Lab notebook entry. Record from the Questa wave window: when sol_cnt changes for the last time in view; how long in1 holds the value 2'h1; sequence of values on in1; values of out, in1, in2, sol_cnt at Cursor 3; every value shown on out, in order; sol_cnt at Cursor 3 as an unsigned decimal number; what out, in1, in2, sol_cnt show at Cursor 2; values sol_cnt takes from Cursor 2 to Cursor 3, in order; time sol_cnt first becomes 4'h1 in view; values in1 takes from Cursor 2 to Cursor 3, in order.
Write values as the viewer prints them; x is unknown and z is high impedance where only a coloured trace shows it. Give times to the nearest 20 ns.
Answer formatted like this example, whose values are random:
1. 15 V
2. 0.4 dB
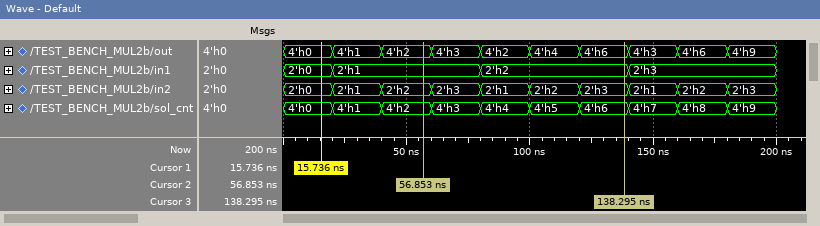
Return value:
1. 180 ns
2. 60 ns
3. 2'h0, 2'h1, 2'h2, 2'h3
4. out=4'h6, in1=2'h2, in2=2'h3, sol_cnt=4'h6
5. 4'h0, 4'h1, 4'h2, 4'h3, 4'h2, 4'h4, 4'h6, 4'h3, 4'h6, 4'h9
6. 6
7. out=4'h2, in1=2'h1, in2=2'h2, sol_cnt=4'h2
8. 4'h2, 4'h3, 4'h4, 4'h5, 4'h6
9. 20 ns
10. 2'h1, 2'h2
